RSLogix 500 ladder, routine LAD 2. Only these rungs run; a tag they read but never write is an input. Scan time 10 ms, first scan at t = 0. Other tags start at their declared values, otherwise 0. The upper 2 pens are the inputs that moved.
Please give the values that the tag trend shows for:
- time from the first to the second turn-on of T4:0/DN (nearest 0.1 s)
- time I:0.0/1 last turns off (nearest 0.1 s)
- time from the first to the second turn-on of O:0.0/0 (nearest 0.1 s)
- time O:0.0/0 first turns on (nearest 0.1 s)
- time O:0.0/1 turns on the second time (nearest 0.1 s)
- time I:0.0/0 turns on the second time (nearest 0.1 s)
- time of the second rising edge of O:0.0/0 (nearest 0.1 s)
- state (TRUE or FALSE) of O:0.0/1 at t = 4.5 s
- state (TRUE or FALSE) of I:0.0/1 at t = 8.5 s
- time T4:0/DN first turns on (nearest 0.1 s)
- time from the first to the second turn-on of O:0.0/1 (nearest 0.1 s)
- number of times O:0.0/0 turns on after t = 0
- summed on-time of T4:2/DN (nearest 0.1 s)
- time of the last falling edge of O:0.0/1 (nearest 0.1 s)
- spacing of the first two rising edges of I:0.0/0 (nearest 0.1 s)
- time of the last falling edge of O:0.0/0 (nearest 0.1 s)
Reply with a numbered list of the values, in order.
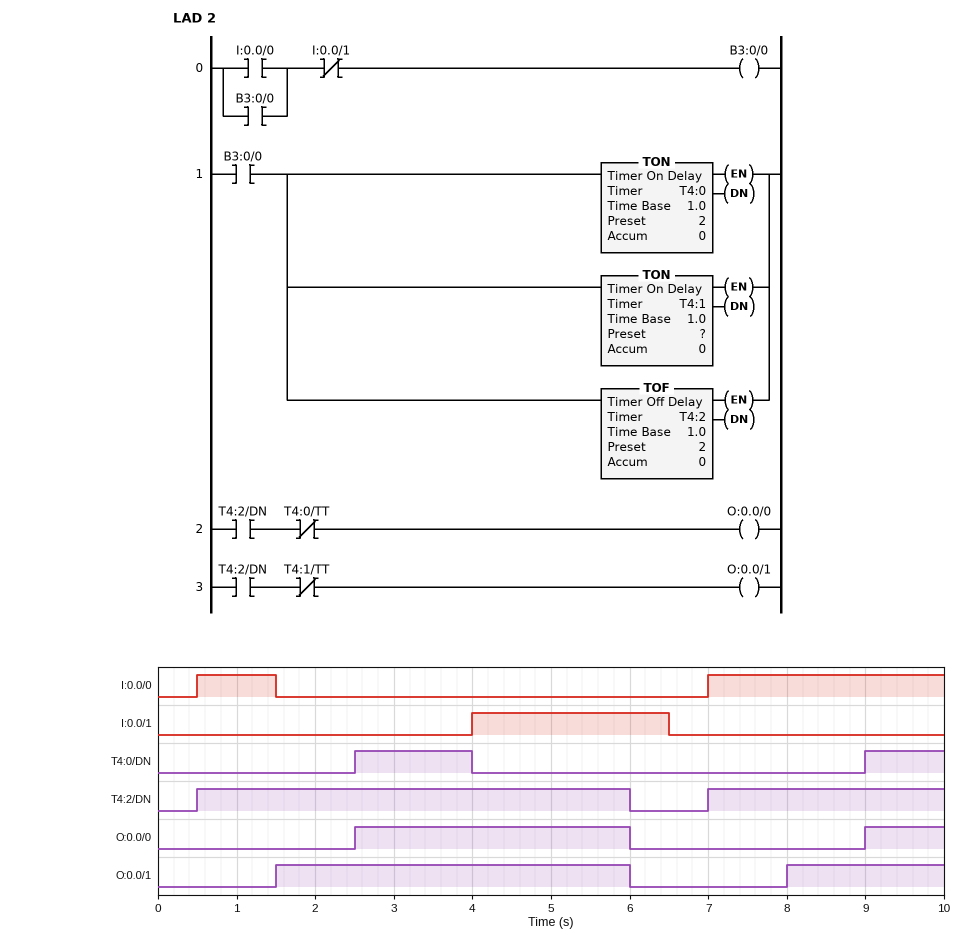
1. 6.5 s
2. 6.5 s
3. 6.5 s
4. 2.5 s
5. 8.0 s
6. 7.0 s
7. 9.0 s
8. TRUE
9. FALSE
10. 2.5 s
11. 6.5 s
12. 2
13. 8.5 s
14. 6.0 s
15. 6.5 s
16. 6.0 s
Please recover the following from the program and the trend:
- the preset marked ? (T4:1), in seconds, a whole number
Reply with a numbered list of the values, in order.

1. 1 s
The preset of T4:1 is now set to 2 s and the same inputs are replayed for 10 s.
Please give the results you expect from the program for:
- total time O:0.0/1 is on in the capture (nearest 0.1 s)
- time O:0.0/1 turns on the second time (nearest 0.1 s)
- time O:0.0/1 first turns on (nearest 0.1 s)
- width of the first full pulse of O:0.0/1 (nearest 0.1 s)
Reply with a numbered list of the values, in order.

1. 4.5 s
2. 9.0 s
3. 2.5 s
4. 3.5 s
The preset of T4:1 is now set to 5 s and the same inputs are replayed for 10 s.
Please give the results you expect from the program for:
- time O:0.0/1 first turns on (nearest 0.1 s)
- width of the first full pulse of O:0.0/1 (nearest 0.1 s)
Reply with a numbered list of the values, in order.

1. 4.0 s
2. 2.0 s
